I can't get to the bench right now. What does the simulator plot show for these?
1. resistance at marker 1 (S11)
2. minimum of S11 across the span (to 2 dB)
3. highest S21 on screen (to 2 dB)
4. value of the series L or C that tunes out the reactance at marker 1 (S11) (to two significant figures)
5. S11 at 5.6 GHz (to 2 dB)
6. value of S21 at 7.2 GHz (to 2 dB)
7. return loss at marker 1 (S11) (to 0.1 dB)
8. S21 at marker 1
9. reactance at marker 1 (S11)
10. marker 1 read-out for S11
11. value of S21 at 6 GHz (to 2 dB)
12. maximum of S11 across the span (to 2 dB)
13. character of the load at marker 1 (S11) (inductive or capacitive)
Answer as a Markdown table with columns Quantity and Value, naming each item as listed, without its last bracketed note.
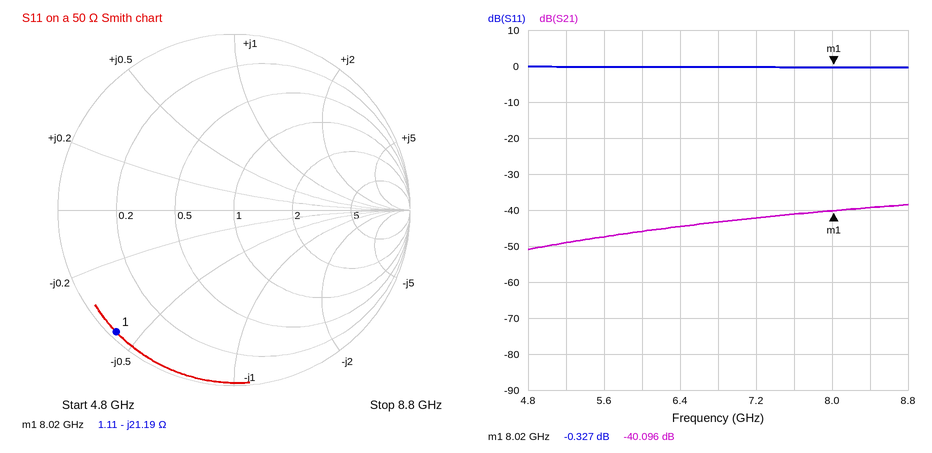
| Quantity | Value |
|---|---|
| resistance at marker 1 | 1.11 Ω |
| minimum of S11 across the span | 0 dB |
| highest S21 on screen | -38 dB |
| value of the series L or C that tunes out the reactance at marker 1 (S11) | 420 pH |
| S11 at 5.6 GHz | 0 dB |
| value of S21 at 7.2 GHz | -42 dB |
| return loss at marker 1 (S11) | 0.3 dB |
| S21 at marker 1 | -40.096 dB |
| reactance at marker 1 | -21.19 Ω |
| marker 1 read-out for S11 | -0.327 dB |
| value of S21 at 6 GHz | -46 dB |
| maximum of S11 across the span | 0 dB |
| character of the load at marker 1 (S11) | capacitive |
